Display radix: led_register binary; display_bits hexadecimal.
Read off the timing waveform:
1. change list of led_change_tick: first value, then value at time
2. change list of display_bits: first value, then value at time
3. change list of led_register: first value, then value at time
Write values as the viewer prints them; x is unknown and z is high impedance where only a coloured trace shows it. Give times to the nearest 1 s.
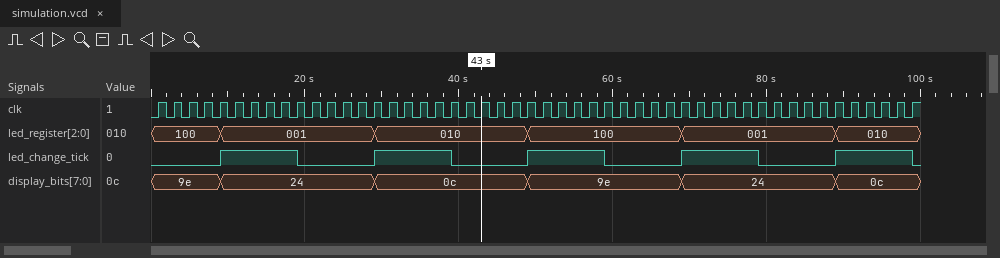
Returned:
0, 1 at 9 s, 0 at 19 s, 1 at 29 s, 0 at 39 s, 1 at 49 s, 0 at 59 s, 1 at 69 s, 0 at 79 s, 1 at 89 s, 0 at 99 s
9e, 24 at 9 s, 0c at 29 s, 9e at 49 s, 24 at 69 s, 0c at 89 s
100, 001 at 9 s, 010 at 29 s, 100 at 49 s, 001 at 69 s, 010 at 89 s
